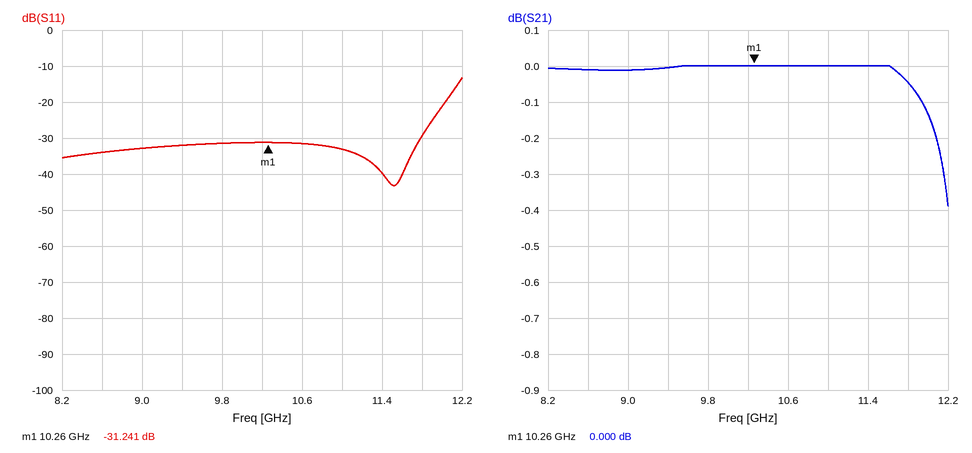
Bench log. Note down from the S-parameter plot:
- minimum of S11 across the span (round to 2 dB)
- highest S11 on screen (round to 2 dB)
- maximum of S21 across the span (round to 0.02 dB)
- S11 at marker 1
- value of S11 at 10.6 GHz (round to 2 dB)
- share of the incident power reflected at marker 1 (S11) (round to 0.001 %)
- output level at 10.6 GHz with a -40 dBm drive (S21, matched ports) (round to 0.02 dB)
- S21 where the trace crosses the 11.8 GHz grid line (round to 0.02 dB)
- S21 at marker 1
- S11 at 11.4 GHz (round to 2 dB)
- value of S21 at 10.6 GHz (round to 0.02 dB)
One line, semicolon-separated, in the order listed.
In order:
-44 dB; -14 dB; 0.00 dB; -31.241 dB; -32 dB; 0.075 %; -40.00 dBm; -0.04 dB; 0.000 dB; -40 dB; 0.00 dB
